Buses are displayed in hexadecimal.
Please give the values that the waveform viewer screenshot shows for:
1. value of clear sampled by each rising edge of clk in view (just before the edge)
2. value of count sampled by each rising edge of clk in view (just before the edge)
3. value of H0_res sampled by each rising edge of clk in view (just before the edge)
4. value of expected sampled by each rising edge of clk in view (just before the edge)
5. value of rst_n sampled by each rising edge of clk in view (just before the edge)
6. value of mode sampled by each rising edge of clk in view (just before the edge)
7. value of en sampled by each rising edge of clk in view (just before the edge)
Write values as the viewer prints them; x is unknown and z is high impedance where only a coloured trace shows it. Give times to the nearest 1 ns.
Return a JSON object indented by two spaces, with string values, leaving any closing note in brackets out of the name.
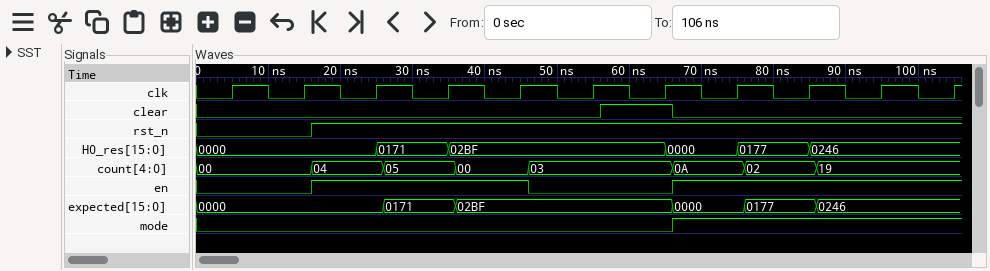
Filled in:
{
  "value of clear sampled by each rising edge of clk in view": "0 0 0 0 0 0 1 0 0 0 0",
  "value of count sampled by each rising edge of clk in view": "00, 00, 04, 05, 00, 03, 03, 0A, 02, 19, 19",
  "value of H0_res sampled by each rising edge of clk in view": "0000, 0000, 0000, 0171, 02BF, 02BF, 02BF, 0000, 0177, 0246, 0246",
  "value of expected sampled by each rising edge of clk in view": "0000, 0000, 0000, 0171, 02BF, 02BF, 02BF, 0000, 0177, 0246, 0246",
  "value of rst_n sampled by each rising edge of clk in view": "0 0 1 1 1 1 1 1 1 1 1",
  "value of mode sampled by each rising edge of clk in view": "0 0 0 0 0 0 0 1 1 1 1",
  "value of en sampled by each rising edge of clk in view": "0 0 1 1 1 0 0 1 1 1 1"
}
